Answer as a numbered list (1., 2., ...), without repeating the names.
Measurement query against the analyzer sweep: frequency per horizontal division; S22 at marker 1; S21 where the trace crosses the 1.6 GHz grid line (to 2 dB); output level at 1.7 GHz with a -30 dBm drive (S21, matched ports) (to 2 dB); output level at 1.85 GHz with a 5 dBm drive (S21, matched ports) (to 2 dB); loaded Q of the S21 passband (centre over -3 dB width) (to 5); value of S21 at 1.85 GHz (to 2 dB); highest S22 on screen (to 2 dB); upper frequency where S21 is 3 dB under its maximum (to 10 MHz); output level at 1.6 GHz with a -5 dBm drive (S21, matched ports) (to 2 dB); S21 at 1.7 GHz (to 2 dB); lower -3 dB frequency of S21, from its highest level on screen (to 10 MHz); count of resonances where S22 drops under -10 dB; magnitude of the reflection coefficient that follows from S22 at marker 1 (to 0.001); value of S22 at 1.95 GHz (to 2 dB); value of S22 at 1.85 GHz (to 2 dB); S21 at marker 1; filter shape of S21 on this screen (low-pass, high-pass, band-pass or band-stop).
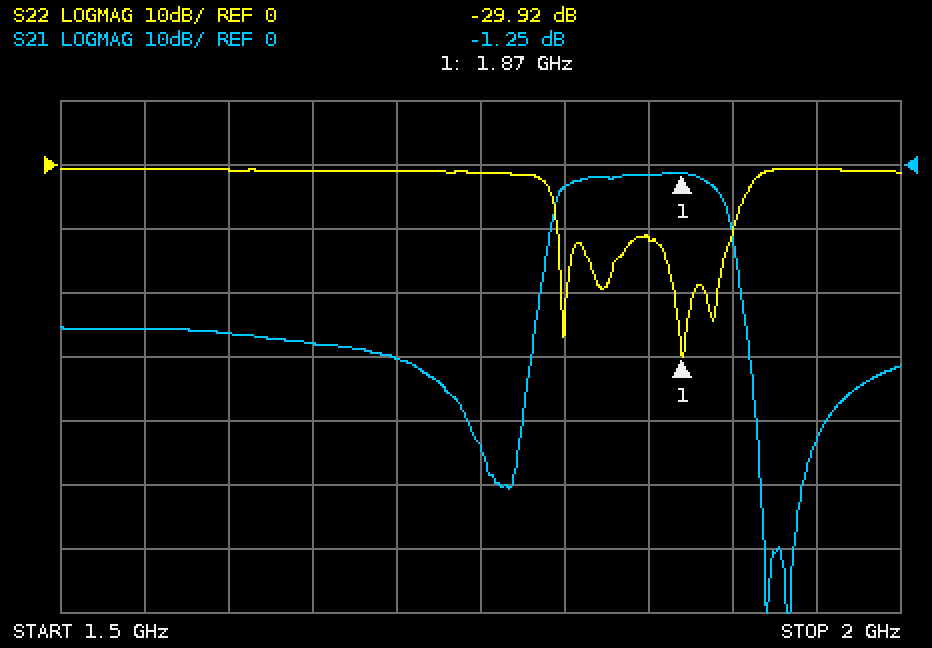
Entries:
1. 50 MHz
2. -29.92 dB
3. -26 dB
4. -60 dBm
5. 4 dBm
6. 20
7. -2 dB
8. 0 dB
9. 1.89 GHz
10. -32 dBm
11. -30 dB
12. 1.80 GHz
13. 4
14. 0.032
15. 0 dB
16. -12 dB
17. -1.25 dB
18. band-pass
